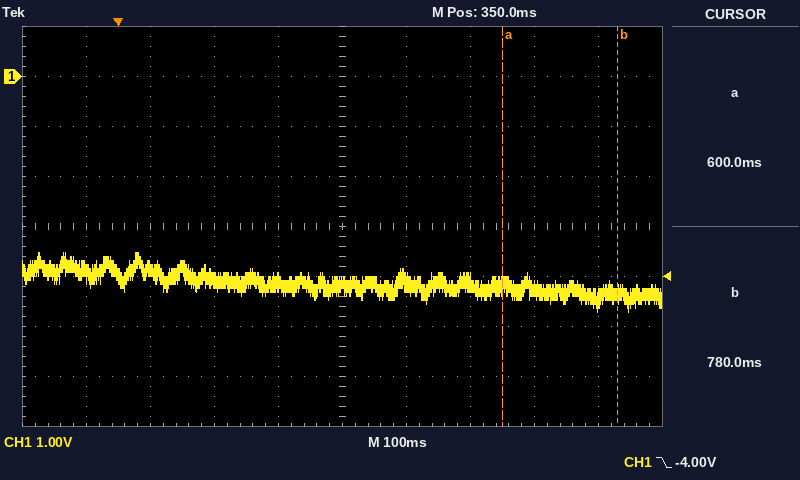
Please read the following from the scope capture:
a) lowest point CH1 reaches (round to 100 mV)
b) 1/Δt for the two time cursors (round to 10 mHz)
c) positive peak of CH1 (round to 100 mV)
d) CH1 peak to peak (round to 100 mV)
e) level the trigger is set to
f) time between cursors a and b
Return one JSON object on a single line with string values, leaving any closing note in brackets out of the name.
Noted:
{"lowest point CH1 reaches": "-4.7 V", "1/Δt for the two time cursors": "5.56 Hz", "positive peak of CH1": "-3.5 V", "CH1 peak to peak": "1.2 V", "level the trigger is set to": "-4.00 V", "time between cursors a and b": "180 ms"}
